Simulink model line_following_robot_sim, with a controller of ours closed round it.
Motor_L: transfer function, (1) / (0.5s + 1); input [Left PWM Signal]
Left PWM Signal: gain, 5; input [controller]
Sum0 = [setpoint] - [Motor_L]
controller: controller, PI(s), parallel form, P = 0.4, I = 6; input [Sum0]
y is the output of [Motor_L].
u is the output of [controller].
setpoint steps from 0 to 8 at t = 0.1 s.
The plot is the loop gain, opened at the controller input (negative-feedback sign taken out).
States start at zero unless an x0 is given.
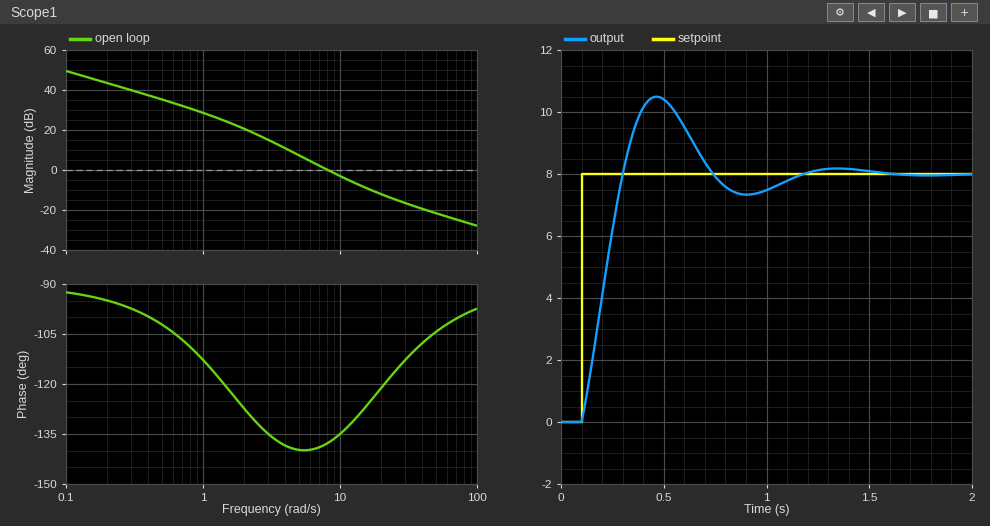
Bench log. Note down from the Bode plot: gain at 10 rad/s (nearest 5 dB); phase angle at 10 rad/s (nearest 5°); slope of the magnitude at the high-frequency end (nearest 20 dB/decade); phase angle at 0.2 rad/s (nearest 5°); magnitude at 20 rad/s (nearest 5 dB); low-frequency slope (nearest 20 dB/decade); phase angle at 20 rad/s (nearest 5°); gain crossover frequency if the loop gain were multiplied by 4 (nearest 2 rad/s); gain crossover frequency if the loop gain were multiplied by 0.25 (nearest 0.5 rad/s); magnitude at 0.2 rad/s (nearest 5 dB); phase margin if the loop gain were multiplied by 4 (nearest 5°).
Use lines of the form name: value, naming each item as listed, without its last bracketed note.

gain at 10 rad/s: -5 dB
phase angle at 10 rad/s: -135°
slope of the magnitude at the high-frequency end: -20 dB/decade
phase angle at 0.2 rad/s: -95°
magnitude at 20 rad/s: -10 dB
low-frequency slope: -20 dB/decade
phase angle at 20 rad/s: -120°
gain crossover frequency if the loop gain were multiplied by 4: 20 rad/s
gain crossover frequency if the loop gain were multiplied by 0.25: 3.5 rad/s
magnitude at 0.2 rad/s: 45 dB
phase margin if the loop gain were multiplied by 4: 60°
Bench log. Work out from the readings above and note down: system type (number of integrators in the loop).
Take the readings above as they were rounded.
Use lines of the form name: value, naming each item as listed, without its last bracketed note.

system type: 1
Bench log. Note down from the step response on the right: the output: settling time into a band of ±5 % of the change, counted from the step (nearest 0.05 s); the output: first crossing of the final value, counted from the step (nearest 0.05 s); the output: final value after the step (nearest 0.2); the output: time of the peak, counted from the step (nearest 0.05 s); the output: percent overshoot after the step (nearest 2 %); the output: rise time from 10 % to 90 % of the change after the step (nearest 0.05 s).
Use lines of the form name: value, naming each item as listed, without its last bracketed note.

the output: settling time into a band of ±5 % of the change, counted from the step: 0.95 s
the output: first crossing of the final value, counted from the step: 0.20 s
the output: final value after the step: 8.0
the output: time of the peak, counted from the step: 0.35 s
the output: percent overshoot after the step: 32 %
the output: rise time from 10 % to 90 % of the change after the step: 0.15 s
